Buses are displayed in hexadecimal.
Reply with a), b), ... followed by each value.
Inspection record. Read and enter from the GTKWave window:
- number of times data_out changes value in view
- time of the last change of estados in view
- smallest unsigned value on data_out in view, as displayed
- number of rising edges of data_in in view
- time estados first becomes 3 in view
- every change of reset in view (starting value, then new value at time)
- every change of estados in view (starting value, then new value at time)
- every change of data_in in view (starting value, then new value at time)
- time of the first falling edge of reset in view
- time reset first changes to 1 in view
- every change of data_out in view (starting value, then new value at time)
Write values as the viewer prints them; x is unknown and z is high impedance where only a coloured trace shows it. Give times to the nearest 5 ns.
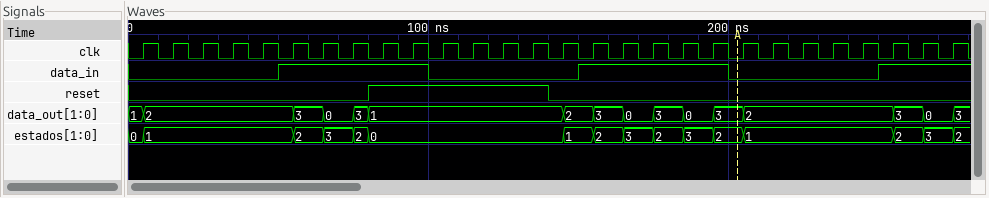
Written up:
a) 15
b) 275 ns
c) 0
d) 3
e) 65 ns
f) 0, 1 at 80 ns, 0 at 140 ns
g) 0, 1 at 5 ns, 2 at 55 ns, 3 at 65 ns, 2 at 75 ns, 0 at 80 ns, 1 at 145 ns, 2 at 155 ns, 3 at 165 ns, 2 at 175 ns, 3 at 185 ns, 2 at 195 ns, 1 at 205 ns, 2 at 255 ns, 3 at 265 ns, 2 at 275 ns
h) 0, 1 at 50 ns, 0 at 100 ns, 1 at 150 ns, 0 at 200 ns, 1 at 250 ns
i) 140 ns
j) 80 ns
k) 1, 2 at 5 ns, 3 at 55 ns, 0 at 65 ns, 3 at 75 ns, 1 at 80 ns, 2 at 145 ns, 3 at 155 ns, 0 at 165 ns, 3 at 175 ns, 0 at 185 ns, 3 at 195 ns, 2 at 205 ns, 3 at 255 ns, 0 at 265 ns, 3 at 275 ns
